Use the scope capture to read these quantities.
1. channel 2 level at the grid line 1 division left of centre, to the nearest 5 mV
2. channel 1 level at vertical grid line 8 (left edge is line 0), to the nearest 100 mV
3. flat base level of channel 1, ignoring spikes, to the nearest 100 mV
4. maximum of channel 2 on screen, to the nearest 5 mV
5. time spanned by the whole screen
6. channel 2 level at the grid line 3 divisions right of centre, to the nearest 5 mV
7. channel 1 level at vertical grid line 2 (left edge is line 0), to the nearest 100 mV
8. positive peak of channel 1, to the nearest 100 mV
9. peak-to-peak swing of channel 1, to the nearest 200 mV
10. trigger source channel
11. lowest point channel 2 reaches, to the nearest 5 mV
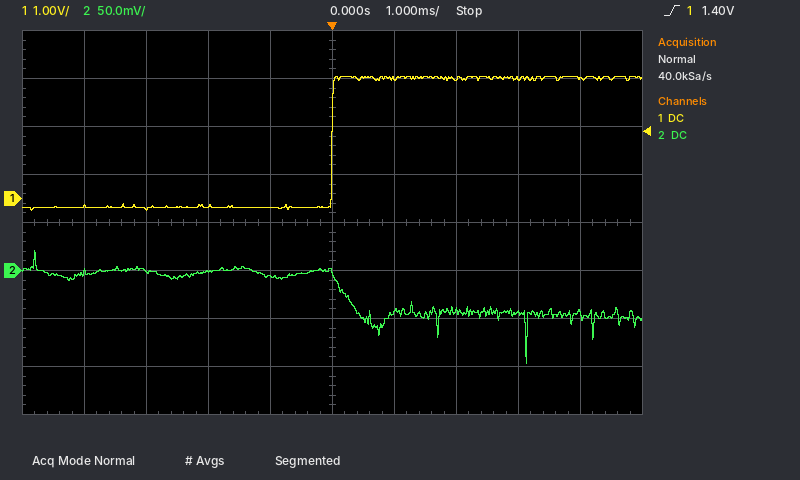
-5 mV
2.5 V
-200 mV
20 mV
10 ms
-45 mV
-200 mV
2.5 V
2.8 V
channel 1
-95 mV
